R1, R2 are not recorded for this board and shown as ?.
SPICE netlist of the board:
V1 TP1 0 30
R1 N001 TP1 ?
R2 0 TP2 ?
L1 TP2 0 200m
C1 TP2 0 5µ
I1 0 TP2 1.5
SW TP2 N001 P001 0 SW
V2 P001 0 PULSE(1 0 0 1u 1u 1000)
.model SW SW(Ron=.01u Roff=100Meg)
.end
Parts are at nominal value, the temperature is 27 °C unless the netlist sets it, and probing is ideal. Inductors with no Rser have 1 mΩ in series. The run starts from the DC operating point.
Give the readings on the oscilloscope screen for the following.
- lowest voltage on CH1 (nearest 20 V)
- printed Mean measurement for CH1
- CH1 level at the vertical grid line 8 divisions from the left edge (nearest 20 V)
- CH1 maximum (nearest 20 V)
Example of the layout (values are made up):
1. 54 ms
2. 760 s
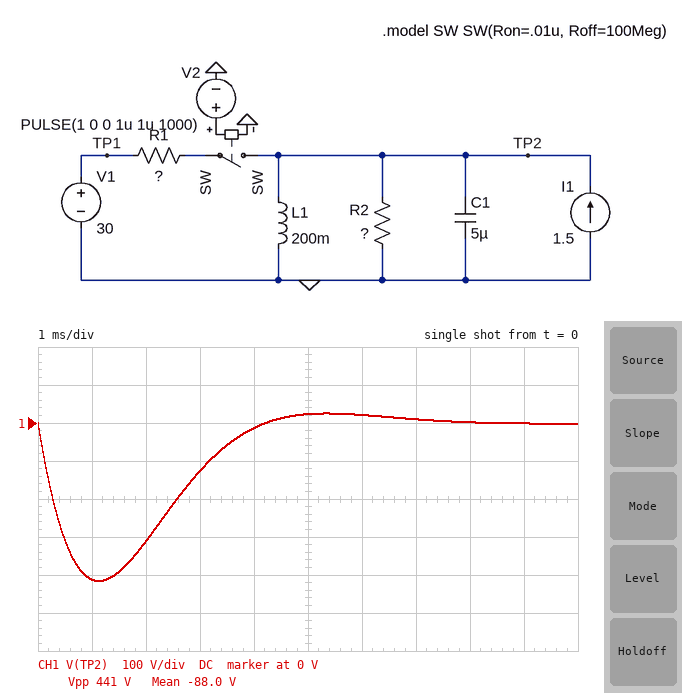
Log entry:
1. -420 V
2. -88.0 V
3. 0 V
4. 20 V
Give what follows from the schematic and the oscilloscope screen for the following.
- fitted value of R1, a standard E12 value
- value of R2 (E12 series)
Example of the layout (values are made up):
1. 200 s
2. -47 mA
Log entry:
1. 6.8 Ω
2. 150 Ω
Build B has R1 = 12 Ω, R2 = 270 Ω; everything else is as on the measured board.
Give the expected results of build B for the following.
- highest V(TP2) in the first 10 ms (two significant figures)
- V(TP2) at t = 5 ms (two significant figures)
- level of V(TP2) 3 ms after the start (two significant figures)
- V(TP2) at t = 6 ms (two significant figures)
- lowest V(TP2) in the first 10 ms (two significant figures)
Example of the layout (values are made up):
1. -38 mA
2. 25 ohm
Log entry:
1. 89 V
2. 84 V
3. -62 V
4. 38 V
5. -310 V
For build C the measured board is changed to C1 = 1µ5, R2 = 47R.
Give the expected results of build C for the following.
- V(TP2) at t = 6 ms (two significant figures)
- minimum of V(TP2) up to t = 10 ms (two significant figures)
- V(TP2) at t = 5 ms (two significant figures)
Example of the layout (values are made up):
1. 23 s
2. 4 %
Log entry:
1. -51 V
2. -200 V
3. -65 V
